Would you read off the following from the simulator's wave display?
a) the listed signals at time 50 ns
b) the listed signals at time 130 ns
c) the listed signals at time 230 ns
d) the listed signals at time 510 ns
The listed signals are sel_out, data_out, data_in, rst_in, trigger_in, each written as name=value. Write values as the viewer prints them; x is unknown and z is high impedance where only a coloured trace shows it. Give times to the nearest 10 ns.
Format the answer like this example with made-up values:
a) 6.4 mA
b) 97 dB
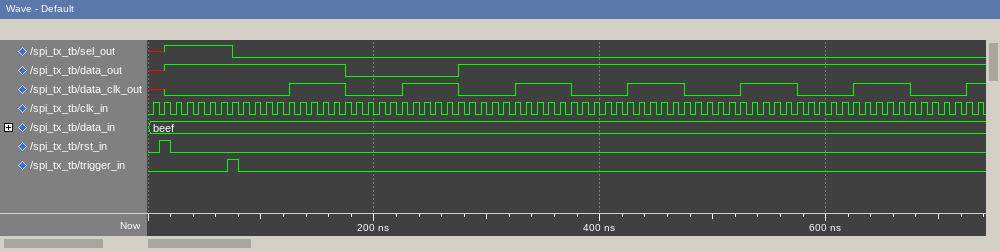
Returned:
a) sel_out=1, data_out=1, data_in=beef, rst_in=0, trigger_in=0
b) sel_out=0, data_out=1, data_in=beef, rst_in=0, trigger_in=0
c) sel_out=0, data_out=0, data_in=beef, rst_in=0, trigger_in=0
d) sel_out=0, data_out=1, data_in=beef, rst_in=0, trigger_in=0
